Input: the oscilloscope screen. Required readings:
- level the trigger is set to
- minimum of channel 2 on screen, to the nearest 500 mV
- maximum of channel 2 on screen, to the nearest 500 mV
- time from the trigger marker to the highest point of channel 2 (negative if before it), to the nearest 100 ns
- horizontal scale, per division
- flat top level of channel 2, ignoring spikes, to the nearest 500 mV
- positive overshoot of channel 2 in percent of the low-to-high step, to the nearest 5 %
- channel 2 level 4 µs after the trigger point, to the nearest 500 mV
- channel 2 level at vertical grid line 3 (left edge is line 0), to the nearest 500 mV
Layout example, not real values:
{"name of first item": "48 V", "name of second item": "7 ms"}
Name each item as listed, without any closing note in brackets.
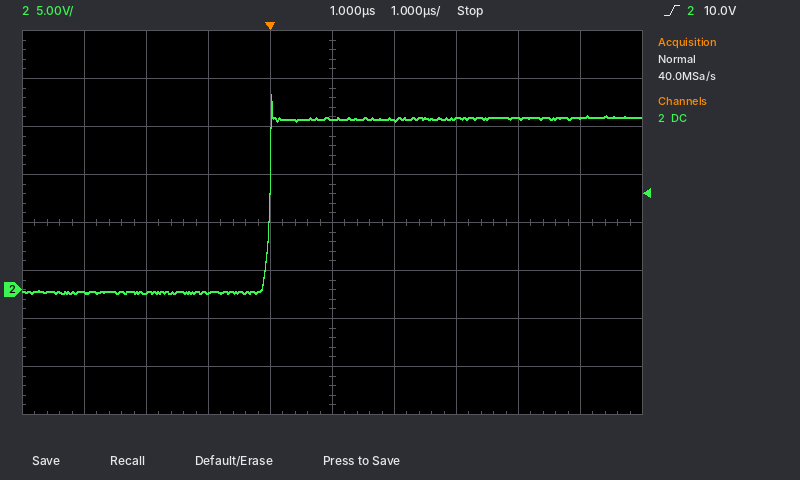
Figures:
{"level the trigger is set to": "10.0 V", "minimum of channel 2 on screen, to the nearest 500 mV": "-500 mV", "maximum of channel 2 on screen, to the nearest 500 mV": "20.5 V", "time from the trigger marker to the highest point of channel 2 (negative if before it), to the nearest 100 ns": "0.0 µs", "horizontal scale, per division": "1 µs", "flat top level of channel 2, ignoring spikes, to the nearest 500 mV": "18.0 V", "positive overshoot of channel 2 in percent of the low-to-high step, to the nearest 5 %": "15 %", "channel 2 level 4 µs after the trigger point, to the nearest 500 mV": "18.0 V", "channel 2 level at vertical grid line 3 (left edge is line 0), to the nearest 500 mV": "-500 mV"}
